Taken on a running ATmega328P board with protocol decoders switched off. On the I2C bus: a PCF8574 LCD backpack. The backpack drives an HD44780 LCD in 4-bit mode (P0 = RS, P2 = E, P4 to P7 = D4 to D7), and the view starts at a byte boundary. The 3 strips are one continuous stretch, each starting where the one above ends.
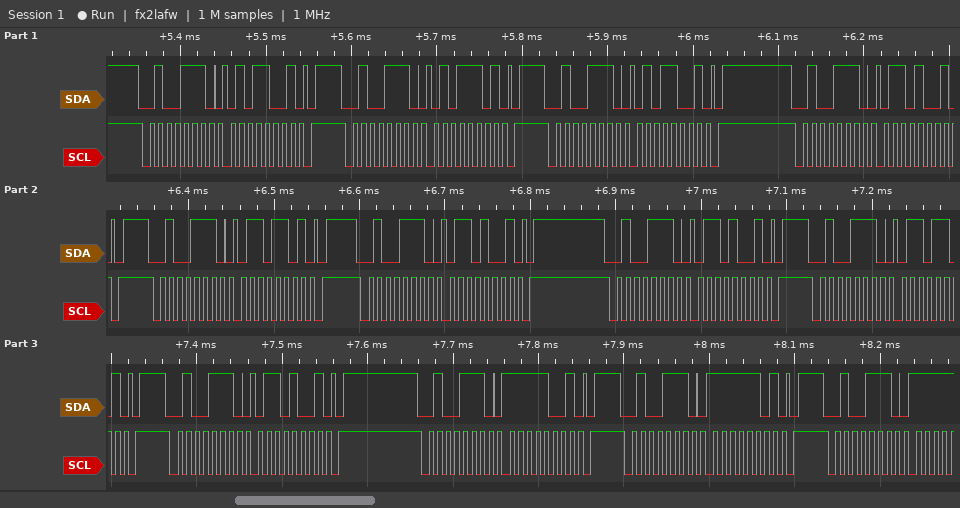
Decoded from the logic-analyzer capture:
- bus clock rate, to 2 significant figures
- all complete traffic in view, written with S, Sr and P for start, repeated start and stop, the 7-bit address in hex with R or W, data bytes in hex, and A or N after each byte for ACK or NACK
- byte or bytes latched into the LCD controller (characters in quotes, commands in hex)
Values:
100 kHz
S 27W A 59 A P S 27W A 5D A P S 27W A 59 A P S 27W A 69 A P S 27W A 6D A P S 27W A 69 A P S 27W A 69 A P S 27W A 6D A P S 27W A 69 A P S 27W A F9 A P S 27W A FD A P S 27W A
'V'
